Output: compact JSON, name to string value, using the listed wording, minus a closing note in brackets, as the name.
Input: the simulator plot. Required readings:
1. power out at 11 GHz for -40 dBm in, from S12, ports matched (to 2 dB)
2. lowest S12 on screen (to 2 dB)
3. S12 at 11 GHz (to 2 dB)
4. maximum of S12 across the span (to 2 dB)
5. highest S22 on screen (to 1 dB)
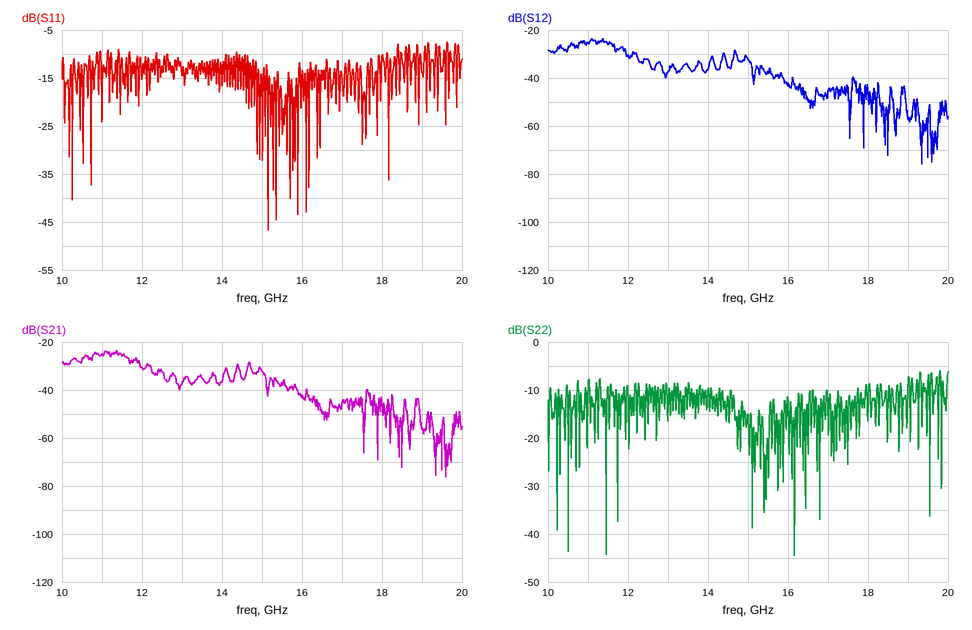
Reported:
{"power out at 11 GHz for -40 dBm in, from S12, ports matched": "-66 dBm", "lowest S12 on screen": "-76 dB", "S12 at 11 GHz": "-26 dB", "maximum of S12 across the span": "-24 dB", "highest S22 on screen": "-6 dB"}
